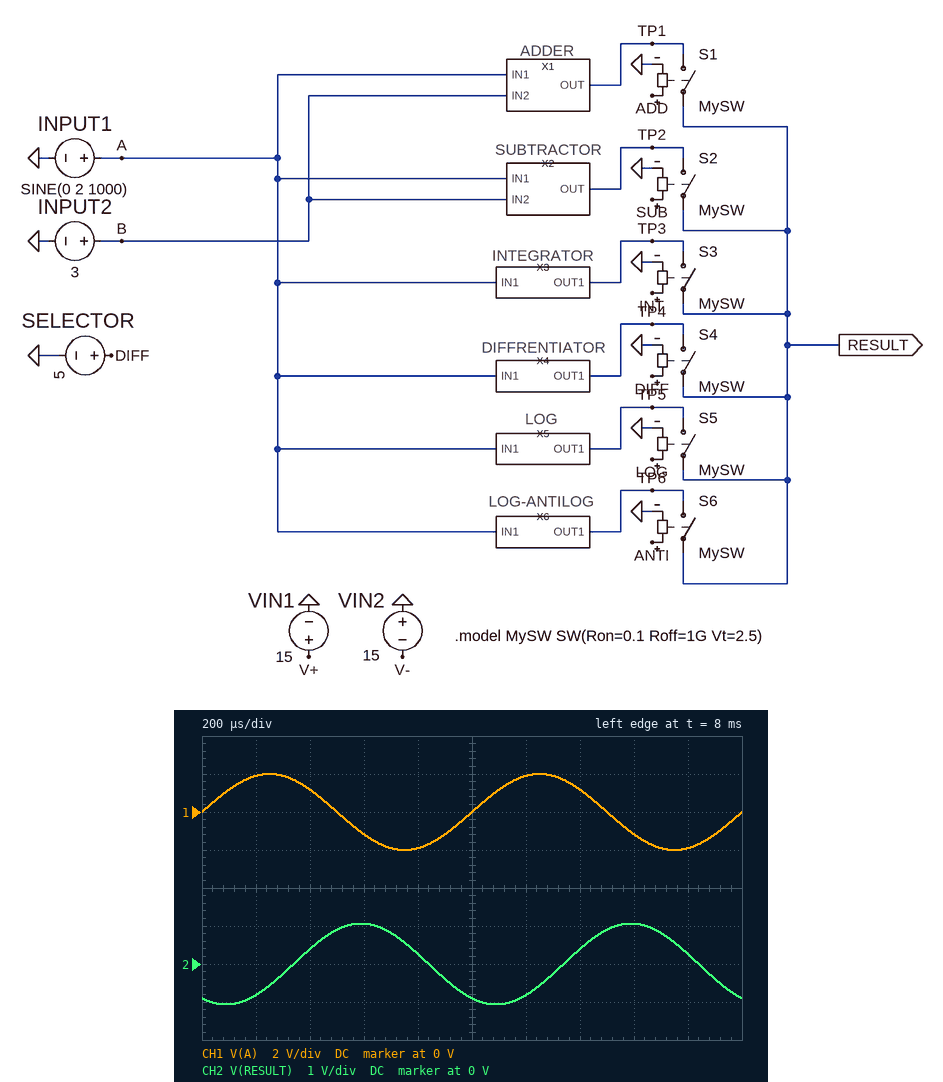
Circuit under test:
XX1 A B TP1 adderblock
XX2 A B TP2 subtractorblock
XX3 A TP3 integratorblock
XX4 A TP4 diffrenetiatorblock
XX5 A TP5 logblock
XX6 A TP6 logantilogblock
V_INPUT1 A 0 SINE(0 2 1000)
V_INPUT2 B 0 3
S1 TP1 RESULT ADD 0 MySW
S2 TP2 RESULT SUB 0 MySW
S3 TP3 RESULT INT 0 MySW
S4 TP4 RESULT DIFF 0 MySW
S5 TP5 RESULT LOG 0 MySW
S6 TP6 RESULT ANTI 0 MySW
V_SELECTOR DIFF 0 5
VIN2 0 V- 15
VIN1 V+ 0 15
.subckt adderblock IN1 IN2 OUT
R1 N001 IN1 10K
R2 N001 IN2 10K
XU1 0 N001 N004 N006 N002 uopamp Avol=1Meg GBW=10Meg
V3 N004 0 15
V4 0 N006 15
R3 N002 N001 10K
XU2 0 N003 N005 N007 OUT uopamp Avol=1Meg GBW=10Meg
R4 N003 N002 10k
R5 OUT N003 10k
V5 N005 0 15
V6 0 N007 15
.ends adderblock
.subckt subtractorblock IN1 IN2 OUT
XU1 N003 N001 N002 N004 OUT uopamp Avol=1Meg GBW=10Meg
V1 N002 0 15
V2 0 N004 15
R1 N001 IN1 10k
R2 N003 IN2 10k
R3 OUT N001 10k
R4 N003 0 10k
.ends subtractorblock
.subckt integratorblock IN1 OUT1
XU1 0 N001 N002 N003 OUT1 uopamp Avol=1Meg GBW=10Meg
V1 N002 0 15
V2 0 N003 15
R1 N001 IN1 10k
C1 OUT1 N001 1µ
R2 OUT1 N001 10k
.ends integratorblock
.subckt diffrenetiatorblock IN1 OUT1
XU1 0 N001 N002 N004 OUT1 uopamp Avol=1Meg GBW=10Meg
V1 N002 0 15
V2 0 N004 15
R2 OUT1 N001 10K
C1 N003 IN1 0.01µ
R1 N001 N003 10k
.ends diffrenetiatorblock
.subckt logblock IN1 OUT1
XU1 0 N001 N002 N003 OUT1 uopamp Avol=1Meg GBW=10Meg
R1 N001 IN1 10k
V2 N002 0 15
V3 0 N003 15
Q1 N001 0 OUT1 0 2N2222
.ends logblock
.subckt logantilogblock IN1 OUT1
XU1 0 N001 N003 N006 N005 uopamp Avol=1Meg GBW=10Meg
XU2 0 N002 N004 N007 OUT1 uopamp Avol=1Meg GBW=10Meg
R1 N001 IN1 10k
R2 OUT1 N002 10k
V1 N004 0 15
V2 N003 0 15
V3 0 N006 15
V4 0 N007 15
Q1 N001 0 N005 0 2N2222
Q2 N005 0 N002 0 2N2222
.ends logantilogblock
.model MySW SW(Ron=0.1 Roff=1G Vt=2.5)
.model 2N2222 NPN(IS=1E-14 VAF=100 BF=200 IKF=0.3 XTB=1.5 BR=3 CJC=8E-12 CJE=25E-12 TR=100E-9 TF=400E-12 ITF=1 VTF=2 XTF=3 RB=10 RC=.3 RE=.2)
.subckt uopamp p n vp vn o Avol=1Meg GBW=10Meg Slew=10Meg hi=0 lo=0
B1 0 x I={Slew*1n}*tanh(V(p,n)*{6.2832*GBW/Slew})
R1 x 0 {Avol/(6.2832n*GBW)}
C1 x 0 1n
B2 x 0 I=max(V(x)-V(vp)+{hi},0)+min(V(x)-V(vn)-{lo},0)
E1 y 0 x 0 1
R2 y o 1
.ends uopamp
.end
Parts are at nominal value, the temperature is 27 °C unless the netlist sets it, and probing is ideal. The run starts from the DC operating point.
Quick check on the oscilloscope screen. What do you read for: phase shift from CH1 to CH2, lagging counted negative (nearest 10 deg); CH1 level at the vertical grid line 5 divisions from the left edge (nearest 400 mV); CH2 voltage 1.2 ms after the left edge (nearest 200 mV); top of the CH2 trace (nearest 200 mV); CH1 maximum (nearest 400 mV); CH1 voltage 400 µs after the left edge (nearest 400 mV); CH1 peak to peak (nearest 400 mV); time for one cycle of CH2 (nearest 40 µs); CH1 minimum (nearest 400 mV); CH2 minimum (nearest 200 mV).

-120 deg
0 V
-800 mV
1.0 V
2.0 V
1.2 V
4.0 V
1.00 ms
-2.0 V
-1.0 V
